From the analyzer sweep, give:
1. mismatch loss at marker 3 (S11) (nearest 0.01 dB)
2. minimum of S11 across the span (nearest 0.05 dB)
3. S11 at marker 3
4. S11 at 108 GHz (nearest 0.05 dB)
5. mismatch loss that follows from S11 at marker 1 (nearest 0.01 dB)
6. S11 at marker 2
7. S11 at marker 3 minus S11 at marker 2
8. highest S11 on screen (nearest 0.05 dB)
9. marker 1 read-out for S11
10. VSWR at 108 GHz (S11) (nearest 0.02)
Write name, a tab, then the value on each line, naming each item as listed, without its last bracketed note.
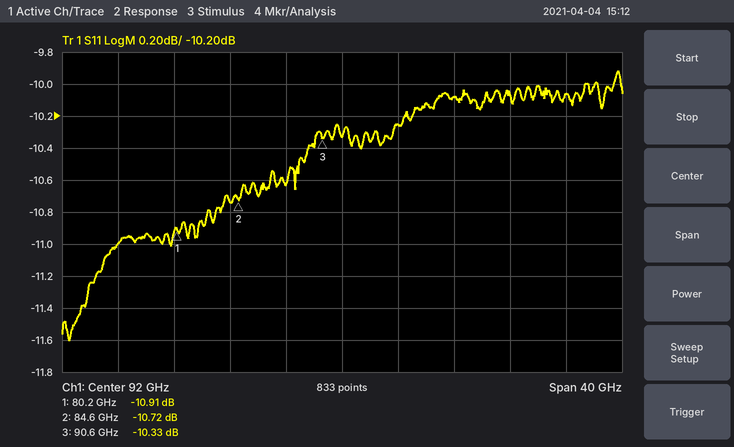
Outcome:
mismatch loss at marker 3 (S11)	0.42 dB
minimum of S11 across the span	-11.60 dB
S11 at marker 3	-10.33 dB
S11 at 108 GHz	-10.05 dB
mismatch loss that follows from S11 at marker 1	0.37 dB
S11 at marker 2	-10.72 dB
S11 at marker 3 minus S11 at marker 2	0.39 dB
highest S11 on screen	-9.90 dB
marker 1 read-out for S11	-10.91 dB
VSWR at 108 GHz (S11)	1.92
